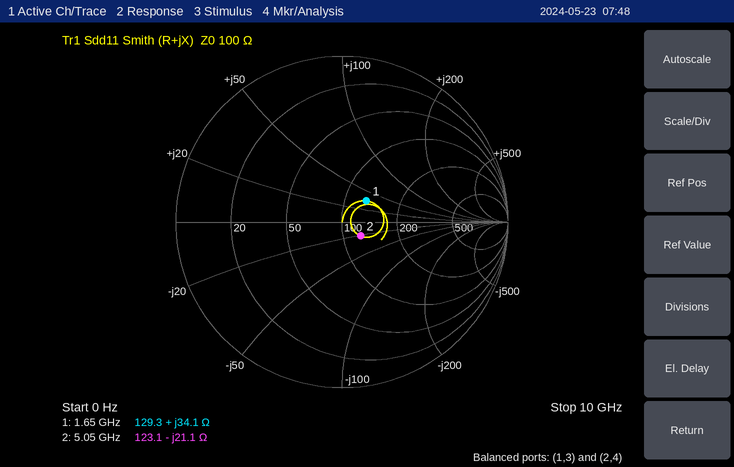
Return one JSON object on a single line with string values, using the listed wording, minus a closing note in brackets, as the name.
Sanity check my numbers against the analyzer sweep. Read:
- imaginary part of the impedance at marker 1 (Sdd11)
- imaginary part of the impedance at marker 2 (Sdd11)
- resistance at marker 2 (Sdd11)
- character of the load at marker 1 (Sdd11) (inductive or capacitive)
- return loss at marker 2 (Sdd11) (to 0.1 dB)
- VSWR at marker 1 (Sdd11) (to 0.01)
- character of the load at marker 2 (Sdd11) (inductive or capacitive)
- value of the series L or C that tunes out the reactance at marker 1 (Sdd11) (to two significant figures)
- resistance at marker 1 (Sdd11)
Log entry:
{"imaginary part of the impedance at marker 1": "+34.1 Ω", "imaginary part of the impedance at marker 2": "-21.1 Ω", "resistance at marker 2": "123.1 Ω", "character of the load at marker 1 (Sdd11)": "inductive", "return loss at marker 2 (Sdd11)": "17.1 dB", "VSWR at marker 1 (Sdd11)": "1.48", "character of the load at marker 2 (Sdd11)": "capacitive", "value of the series L or C that tunes out the reactance at marker 1 (Sdd11)": "2.8 pF", "resistance at marker 1": "129.3 Ω"}
